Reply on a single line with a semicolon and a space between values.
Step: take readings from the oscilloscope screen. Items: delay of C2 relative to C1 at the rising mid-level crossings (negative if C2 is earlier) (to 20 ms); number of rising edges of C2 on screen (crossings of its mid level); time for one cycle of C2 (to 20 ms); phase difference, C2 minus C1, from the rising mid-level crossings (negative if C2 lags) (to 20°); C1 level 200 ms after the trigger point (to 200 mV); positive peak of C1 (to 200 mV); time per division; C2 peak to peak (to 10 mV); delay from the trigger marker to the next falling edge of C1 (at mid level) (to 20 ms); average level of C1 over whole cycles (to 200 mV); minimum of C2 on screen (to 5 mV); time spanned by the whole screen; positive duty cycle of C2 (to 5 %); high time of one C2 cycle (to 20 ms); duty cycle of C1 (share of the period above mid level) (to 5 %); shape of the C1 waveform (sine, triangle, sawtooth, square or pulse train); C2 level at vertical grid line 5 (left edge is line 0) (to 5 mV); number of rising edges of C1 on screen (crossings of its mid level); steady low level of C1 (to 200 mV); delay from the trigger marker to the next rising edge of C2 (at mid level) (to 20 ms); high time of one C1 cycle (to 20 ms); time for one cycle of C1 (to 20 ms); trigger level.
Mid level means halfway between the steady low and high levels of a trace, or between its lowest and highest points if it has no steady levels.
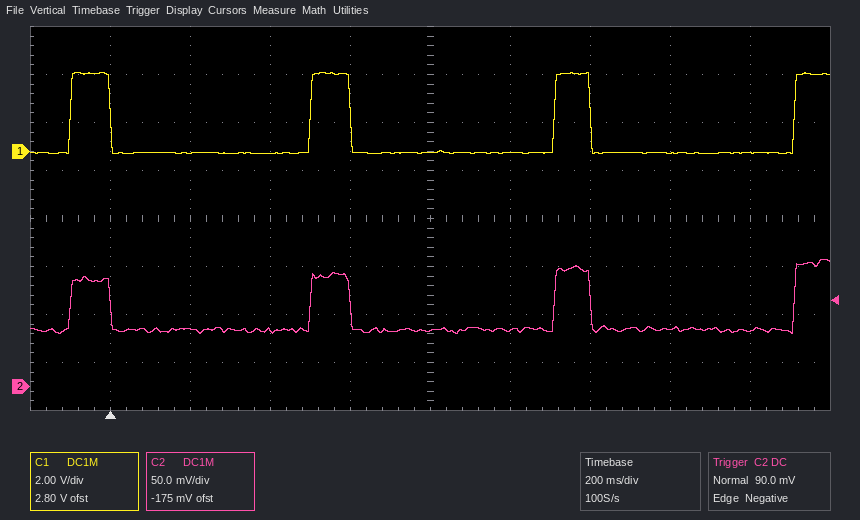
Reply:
0 ms; 4; 600 ms; 0°; 0.0 V; 3.2 V; 200 ms; 80 mV; 600 ms; 400 mV; 55 mV; 2 s; 15 %; 100 ms; 15 %; pulse train; 60 mV; 4; 0.0 V; 500 ms; 100 ms; 600 ms; 90.0 mV
